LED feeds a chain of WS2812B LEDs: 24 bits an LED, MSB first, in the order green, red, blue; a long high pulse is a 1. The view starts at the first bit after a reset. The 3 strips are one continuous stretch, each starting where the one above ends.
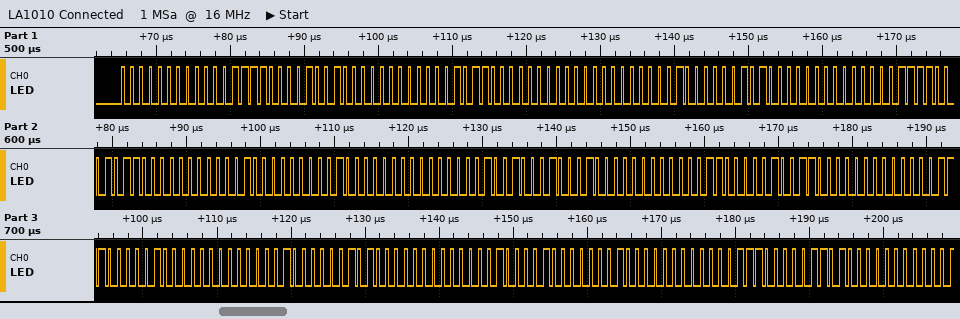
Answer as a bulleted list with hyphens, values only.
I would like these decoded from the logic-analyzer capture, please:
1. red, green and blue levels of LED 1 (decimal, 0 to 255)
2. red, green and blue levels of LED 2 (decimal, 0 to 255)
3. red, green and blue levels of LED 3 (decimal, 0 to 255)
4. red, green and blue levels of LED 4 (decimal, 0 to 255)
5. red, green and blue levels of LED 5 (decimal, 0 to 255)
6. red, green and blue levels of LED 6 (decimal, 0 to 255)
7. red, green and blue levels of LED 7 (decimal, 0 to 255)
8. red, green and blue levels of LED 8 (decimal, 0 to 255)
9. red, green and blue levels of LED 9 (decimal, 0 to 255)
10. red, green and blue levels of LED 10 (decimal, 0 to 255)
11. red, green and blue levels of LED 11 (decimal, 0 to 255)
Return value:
- 15, 0, 9
- 11, 0, 0
- 8, 0, 20
- 15, 0, 22
- 32, 0, 8
- 9, 0, 17
- 12, 0, 19
- 7, 0, 4
- 16, 0, 40
- 33, 0, 1
- 14, 0, 13
